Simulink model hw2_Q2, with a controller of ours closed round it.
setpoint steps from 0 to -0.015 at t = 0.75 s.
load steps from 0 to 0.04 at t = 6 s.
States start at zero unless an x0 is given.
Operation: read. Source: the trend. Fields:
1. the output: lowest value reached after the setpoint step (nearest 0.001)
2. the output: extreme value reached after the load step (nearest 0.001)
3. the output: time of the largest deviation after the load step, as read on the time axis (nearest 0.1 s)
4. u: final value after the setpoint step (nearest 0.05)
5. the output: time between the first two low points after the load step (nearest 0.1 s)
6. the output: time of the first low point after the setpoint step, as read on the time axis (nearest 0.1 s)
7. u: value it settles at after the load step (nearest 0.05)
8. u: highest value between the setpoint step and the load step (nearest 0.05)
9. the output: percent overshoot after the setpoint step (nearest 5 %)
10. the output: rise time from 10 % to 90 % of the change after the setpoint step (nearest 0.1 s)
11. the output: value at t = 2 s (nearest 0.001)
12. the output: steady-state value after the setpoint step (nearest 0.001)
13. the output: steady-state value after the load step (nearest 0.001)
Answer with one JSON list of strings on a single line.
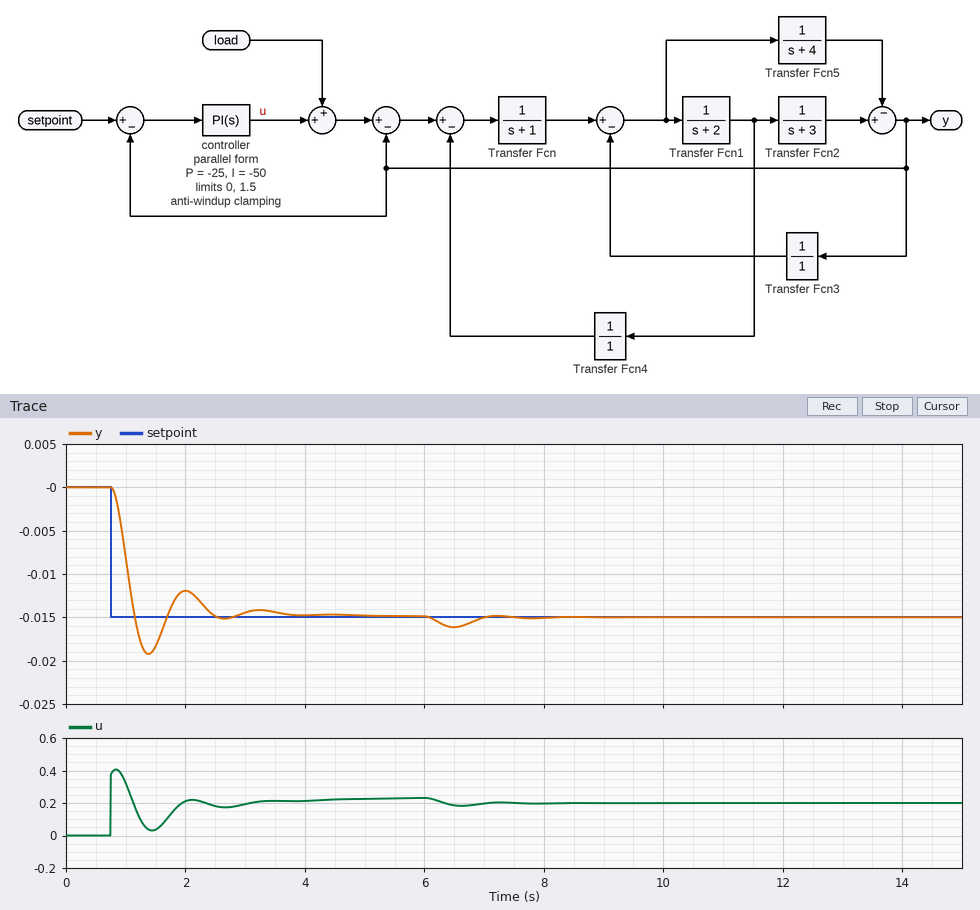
["-0.019", "-0.016", "6.5 s", "0.25", "1.3 s", "1.4 s", "0.20", "0.40", "30 %", "0.3 s", "-0.012", "-0.015", "-0.015"]
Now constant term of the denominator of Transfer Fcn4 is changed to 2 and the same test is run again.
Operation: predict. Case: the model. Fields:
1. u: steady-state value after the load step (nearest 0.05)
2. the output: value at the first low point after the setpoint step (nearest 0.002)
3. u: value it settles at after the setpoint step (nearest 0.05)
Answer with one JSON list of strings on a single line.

["0.15", "-0.020", "0.20"]
